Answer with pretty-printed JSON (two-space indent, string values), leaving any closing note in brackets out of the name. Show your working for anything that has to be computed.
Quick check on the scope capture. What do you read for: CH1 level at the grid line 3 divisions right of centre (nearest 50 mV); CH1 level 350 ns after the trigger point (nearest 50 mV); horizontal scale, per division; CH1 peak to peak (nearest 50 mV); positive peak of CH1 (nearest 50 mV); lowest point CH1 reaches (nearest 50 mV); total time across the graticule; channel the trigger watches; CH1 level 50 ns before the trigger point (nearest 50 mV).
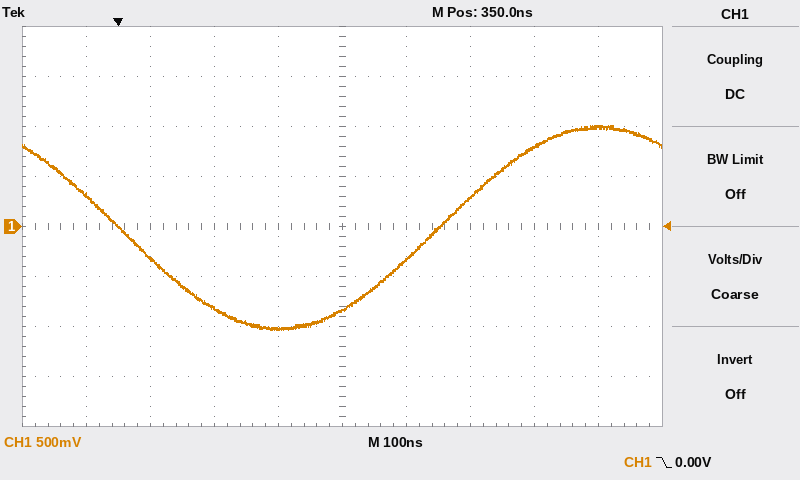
{
  "CH1 level at the grid line 3 divisions right of centre": "800 mV",
  "CH1 level 350 ns after the trigger point": "-850 mV",
  "horizontal scale, per division": "100 ns",
  "CH1 peak to peak": "1.00 V − (-1.05 V) = 2.05 V",
  "positive peak of CH1": "1.00 V",
  "lowest point CH1 reaches": "-1.05 V",
  "total time across the graticule": "1 µs",
  "channel the trigger watches": "CH1",
  "CH1 level 50 ns before the trigger point": "300 mV"
}
